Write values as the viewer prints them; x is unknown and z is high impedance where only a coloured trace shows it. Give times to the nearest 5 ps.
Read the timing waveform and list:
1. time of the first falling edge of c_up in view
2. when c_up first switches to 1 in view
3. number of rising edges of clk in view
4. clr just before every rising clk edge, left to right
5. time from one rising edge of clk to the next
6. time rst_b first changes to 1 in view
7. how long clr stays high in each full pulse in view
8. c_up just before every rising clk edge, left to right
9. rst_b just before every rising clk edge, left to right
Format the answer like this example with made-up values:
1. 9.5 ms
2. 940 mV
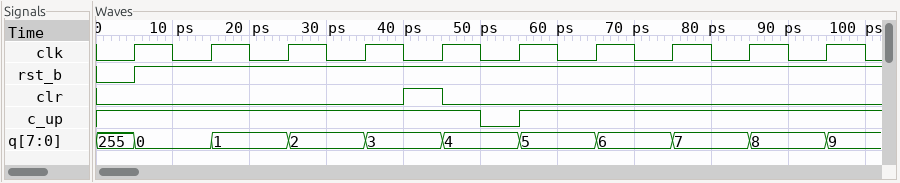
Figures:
1. 50 ps
2. 55 ps
3. 10
4. 0 0 0 0 1 0 0 0 0 0
5. 10 ps
6. 5 ps
7. 5 ps
8. 1 1 1 1 1 0 1 1 1 1
9. 0 1 1 1 1 1 1 1 1 1
